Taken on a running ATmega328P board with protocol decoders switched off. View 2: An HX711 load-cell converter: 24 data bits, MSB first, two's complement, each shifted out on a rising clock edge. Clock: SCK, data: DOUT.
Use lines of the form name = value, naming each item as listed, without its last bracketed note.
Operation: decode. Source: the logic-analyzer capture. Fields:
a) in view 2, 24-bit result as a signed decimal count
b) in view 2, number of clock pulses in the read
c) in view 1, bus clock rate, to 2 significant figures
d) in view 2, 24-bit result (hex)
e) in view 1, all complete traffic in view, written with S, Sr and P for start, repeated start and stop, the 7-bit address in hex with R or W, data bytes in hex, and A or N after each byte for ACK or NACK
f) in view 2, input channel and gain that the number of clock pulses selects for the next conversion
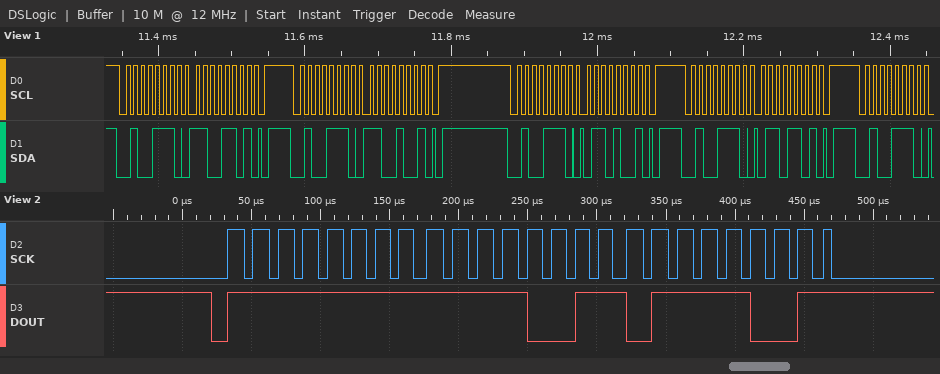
in view 2, 24-bit result as a signed decimal count = -3207
in view 2, number of clock pulses in the read = 25
in view 1, bus clock rate, to 2 significant figures = 100 kHz
in view 2, 24-bit result = 0xFFF379
in view 1, all complete traffic in view, written with S, Sr and P for start, repeated start and stop, the 7-bit address in hex with R or W, data bytes in hex, and A or N after each byte for ACK or NACK = S 27W A CD A P S 27W A C9 A P S 27W A 69 A P S 27W A 6D A P S 27W A
in view 2, input channel and gain that the number of clock pulses selects for the next conversion = channel A, gain 128
